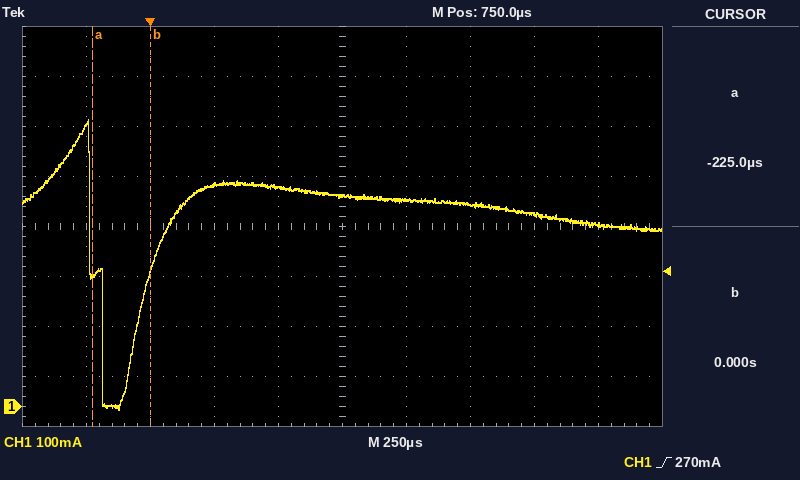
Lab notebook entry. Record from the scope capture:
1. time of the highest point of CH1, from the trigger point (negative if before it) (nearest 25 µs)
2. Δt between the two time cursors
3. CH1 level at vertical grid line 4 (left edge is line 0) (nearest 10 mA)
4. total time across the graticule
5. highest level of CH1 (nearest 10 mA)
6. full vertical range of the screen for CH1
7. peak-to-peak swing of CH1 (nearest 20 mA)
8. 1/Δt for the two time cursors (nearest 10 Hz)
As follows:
-250 µs
225 µs
440 mA
2.5 ms
570 mA
800 mA
580 mA
4.44 kHz
